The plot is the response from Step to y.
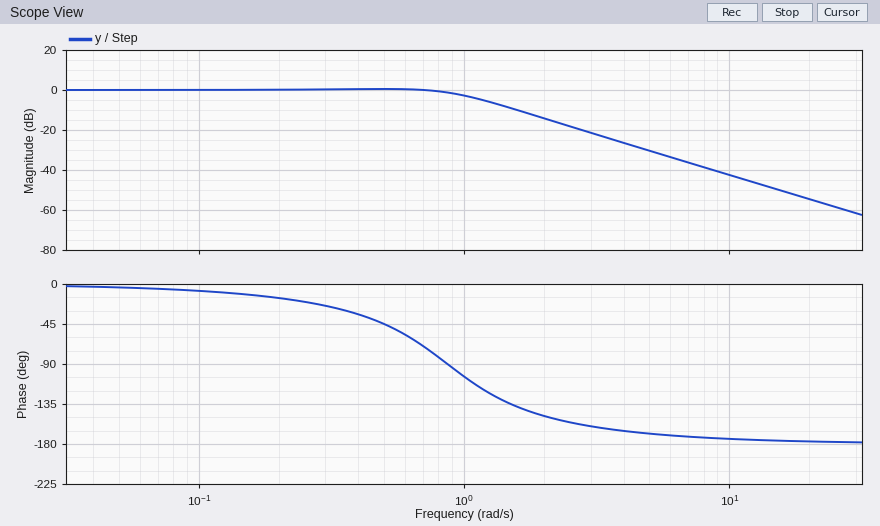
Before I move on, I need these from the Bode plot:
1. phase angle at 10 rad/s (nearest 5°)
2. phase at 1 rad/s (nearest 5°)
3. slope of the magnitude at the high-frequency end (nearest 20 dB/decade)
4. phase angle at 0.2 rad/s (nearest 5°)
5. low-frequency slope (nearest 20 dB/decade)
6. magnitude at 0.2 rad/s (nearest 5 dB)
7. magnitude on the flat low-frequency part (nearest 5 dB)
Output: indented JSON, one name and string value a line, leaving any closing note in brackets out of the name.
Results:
{
  "phase angle at 10 rad/s": "-175°",
  "phase at 1 rad/s": "-105°",
  "slope of the magnitude at the high-frequency end": "-40 dB/decade",
  "phase angle at 0.2 rad/s": "-15°",
  "low-frequency slope": "0 dB/decade",
  "magnitude at 0.2 rad/s": "0 dB",
  "magnitude on the flat low-frequency part": "0 dB"
}
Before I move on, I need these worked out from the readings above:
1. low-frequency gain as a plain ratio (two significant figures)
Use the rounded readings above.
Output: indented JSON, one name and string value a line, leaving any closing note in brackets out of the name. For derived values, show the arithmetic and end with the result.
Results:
{
  "low-frequency gain as a plain ratio": "10^(0 / 20) = 1.0"
}
